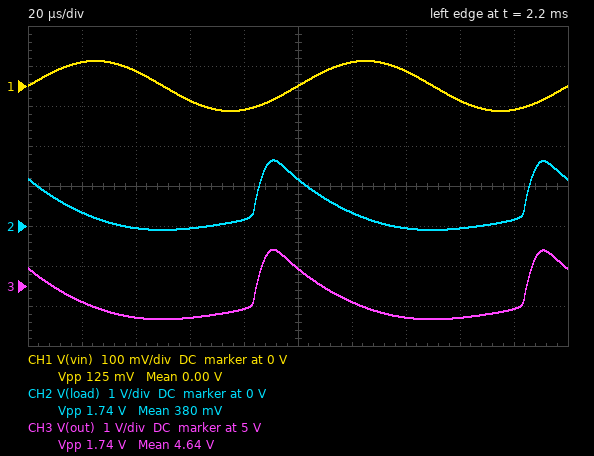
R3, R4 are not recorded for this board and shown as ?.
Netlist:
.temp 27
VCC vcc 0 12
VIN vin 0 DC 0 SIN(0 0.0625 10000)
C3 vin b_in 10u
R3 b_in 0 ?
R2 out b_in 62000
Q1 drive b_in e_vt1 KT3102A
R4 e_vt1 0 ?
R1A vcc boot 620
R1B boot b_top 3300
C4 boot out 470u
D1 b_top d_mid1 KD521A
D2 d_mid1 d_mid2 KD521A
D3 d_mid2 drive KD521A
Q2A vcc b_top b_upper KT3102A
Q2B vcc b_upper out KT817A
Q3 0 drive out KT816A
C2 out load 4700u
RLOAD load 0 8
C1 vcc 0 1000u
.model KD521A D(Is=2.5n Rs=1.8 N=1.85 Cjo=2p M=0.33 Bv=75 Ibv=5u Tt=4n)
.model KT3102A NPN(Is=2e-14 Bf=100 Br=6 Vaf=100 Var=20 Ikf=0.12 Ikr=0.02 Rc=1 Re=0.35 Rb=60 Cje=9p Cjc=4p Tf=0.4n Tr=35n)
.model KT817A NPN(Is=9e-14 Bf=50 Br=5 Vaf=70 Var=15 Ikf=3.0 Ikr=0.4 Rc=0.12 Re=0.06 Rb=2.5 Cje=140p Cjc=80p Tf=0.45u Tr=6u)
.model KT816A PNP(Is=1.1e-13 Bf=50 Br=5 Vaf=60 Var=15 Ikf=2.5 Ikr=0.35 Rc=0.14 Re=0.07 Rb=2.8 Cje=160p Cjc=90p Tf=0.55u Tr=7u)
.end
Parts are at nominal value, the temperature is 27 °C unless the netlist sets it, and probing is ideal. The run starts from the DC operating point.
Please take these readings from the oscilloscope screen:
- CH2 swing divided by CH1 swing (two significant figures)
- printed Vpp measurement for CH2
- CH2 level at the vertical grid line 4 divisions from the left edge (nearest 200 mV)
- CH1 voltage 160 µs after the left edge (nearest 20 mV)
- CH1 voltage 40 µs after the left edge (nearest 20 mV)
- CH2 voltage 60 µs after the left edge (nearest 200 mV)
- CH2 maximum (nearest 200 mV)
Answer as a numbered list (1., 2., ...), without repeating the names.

1. 14
2. 1.74 V
3. 200 mV
4. -40 mV
5. 40 mV
6. 0 V
7. 1.6 V
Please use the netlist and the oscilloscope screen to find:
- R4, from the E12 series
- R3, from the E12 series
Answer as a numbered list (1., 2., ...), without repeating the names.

1. 68 Ω
2. 22 kΩ
